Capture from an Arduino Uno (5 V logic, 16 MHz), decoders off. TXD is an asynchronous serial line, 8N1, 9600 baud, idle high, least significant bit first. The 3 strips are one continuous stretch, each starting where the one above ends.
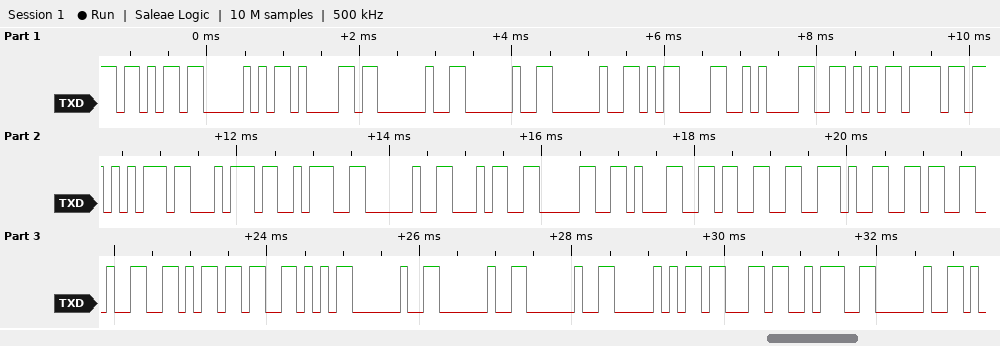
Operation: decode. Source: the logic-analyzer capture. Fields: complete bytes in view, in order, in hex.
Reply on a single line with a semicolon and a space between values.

0x6B 0x50 0x61 0x20 0x20 0x20 0x0D 0x0A 0x56 0x6F 0x75 0x74 0x3A 0x20 0x34 0x30 0x31 0x33 0x2E 0x36 0x32 0x6D 0x56 0x20 0x20 0x20 0x50 0x63 0x3A 0x20
